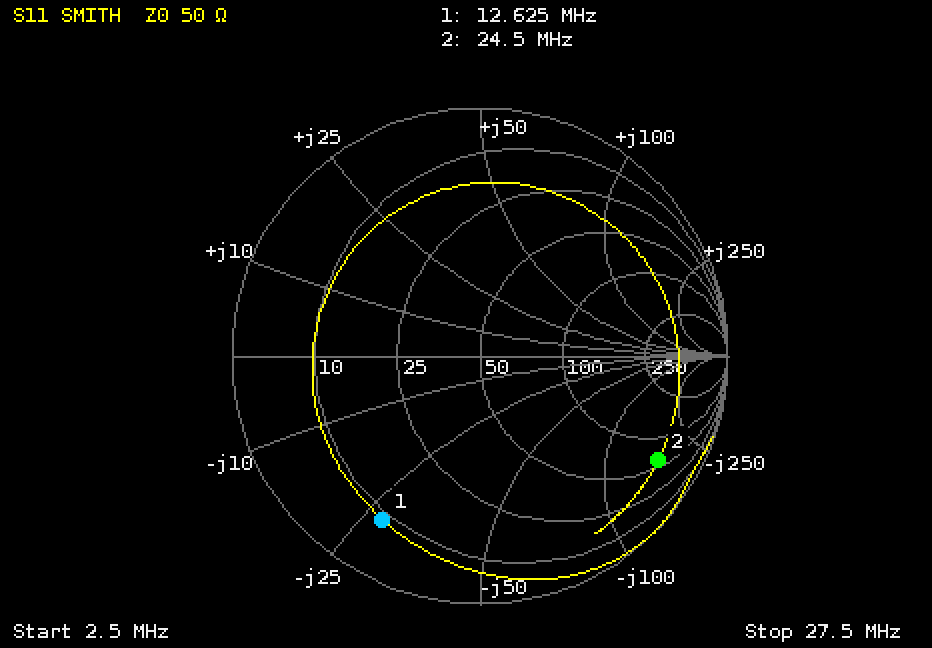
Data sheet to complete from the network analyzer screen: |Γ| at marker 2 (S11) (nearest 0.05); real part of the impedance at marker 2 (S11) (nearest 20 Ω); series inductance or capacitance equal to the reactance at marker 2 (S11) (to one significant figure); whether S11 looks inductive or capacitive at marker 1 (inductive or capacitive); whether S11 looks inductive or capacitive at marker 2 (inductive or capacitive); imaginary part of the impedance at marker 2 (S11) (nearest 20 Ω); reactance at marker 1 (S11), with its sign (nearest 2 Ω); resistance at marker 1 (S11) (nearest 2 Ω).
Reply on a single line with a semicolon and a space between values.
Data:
0.85; 60 Ω; 40 pF; capacitive; capacitive; -160 Ω; -28 Ω; 8 Ω
